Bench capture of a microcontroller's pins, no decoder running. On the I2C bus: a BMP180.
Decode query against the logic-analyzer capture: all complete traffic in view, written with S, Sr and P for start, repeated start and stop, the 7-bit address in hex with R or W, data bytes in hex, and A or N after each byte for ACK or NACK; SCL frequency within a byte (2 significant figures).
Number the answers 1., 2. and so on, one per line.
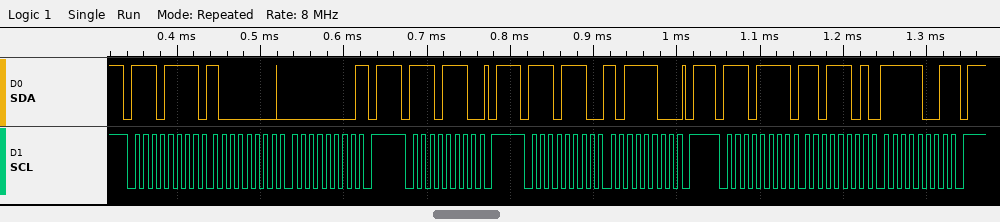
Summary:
1. S 77R A 80 A 00 N P S 77W A P S 77W A BC A P S 77R A DD A F9 N P
2. 100 kHz
